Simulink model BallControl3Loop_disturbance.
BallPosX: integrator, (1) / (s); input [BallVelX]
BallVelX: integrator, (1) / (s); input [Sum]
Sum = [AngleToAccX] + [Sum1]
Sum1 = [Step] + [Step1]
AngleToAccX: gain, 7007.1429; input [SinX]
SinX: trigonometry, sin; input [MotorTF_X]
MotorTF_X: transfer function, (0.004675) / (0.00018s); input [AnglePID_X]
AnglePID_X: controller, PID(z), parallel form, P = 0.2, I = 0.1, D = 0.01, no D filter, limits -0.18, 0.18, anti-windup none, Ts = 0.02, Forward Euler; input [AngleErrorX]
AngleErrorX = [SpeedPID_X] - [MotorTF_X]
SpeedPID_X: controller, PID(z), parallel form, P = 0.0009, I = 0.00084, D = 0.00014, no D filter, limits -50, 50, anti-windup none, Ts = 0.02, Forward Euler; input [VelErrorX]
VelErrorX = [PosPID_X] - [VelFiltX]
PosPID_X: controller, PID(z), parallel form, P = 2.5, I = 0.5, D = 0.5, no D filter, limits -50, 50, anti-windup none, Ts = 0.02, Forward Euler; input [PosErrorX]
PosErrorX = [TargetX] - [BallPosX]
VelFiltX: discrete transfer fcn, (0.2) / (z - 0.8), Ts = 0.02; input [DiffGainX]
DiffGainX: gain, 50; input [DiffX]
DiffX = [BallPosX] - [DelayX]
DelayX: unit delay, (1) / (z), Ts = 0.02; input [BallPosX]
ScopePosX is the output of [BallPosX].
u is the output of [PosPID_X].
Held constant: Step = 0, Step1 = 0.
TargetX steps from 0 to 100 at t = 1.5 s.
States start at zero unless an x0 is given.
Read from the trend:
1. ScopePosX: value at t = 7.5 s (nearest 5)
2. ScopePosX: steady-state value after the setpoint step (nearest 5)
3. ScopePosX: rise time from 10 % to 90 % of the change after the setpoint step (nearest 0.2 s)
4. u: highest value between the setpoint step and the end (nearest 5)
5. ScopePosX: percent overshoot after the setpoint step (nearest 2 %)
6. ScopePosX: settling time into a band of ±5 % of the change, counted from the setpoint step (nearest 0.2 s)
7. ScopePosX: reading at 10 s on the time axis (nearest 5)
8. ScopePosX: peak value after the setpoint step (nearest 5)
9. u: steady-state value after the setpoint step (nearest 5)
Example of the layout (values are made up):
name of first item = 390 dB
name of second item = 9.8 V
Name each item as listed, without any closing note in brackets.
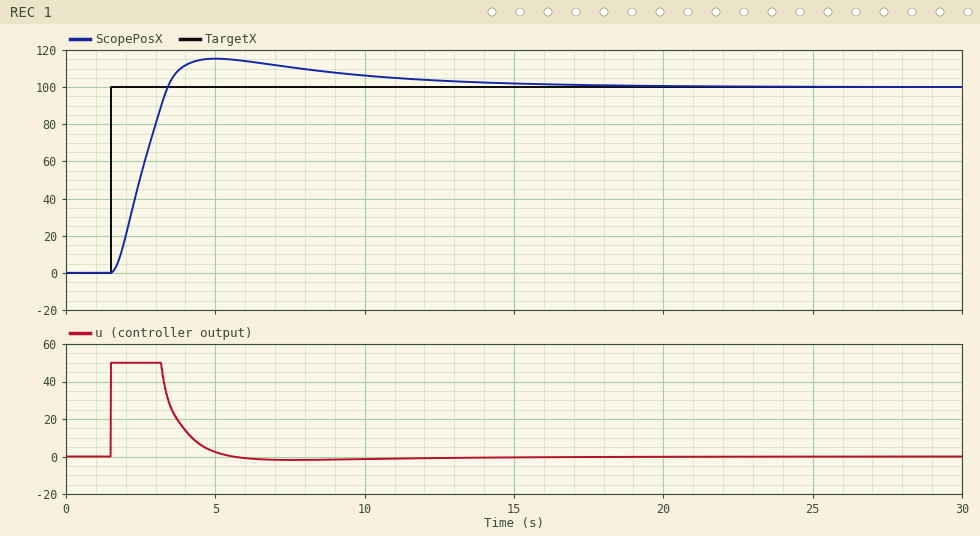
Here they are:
ScopePosX: value at t = 7.5 s = 110
ScopePosX: steady-state value after the setpoint step = 100
ScopePosX: rise time from 10 % to 90 % of the change after the setpoint step = 1.4 s
u: highest value between the setpoint step and the end = 50
ScopePosX: percent overshoot after the setpoint step = 16 %
ScopePosX: settling time into a band of ±5 % of the change, counted from the setpoint step = 9.4 s
ScopePosX: reading at 10 s on the time axis = 105
ScopePosX: peak value after the setpoint step = 115
u: steady-state value after the setpoint step = 0
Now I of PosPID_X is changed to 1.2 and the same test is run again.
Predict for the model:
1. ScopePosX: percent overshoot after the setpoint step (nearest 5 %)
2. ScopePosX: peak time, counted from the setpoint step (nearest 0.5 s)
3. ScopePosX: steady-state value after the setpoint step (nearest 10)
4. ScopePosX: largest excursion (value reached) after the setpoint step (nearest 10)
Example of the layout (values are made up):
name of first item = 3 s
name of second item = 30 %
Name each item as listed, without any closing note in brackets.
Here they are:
ScopePosX: percent overshoot after the setpoint step = 35 %
ScopePosX: peak time, counted from the setpoint step = 3.0 s
ScopePosX: steady-state value after the setpoint step = 100
ScopePosX: largest excursion (value reached) after the setpoint step = 130
